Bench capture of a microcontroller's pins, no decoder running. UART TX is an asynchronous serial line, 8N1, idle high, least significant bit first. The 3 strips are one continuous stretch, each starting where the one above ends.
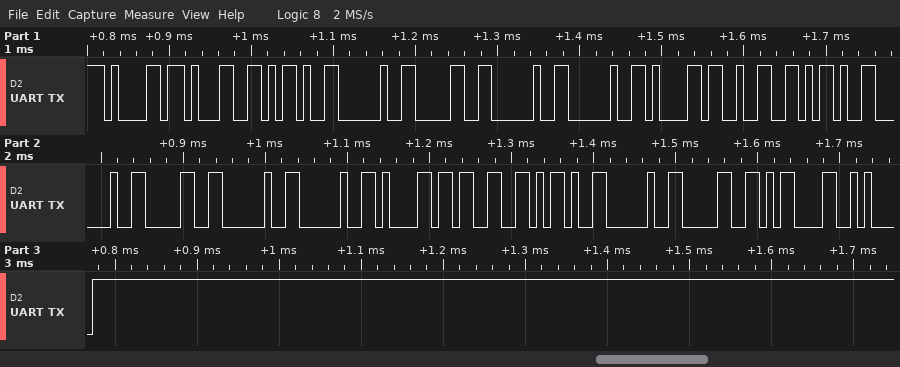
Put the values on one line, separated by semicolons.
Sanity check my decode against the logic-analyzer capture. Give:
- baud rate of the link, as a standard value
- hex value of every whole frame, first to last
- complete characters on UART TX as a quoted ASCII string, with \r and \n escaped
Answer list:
115200 baud; 61 31 2D 20 30 20 20 61 32 2D 20 30 20 20 61 33 2D 20 30 0D 0A; "a1- 0  a2- 0  a3- 0\r\n"
